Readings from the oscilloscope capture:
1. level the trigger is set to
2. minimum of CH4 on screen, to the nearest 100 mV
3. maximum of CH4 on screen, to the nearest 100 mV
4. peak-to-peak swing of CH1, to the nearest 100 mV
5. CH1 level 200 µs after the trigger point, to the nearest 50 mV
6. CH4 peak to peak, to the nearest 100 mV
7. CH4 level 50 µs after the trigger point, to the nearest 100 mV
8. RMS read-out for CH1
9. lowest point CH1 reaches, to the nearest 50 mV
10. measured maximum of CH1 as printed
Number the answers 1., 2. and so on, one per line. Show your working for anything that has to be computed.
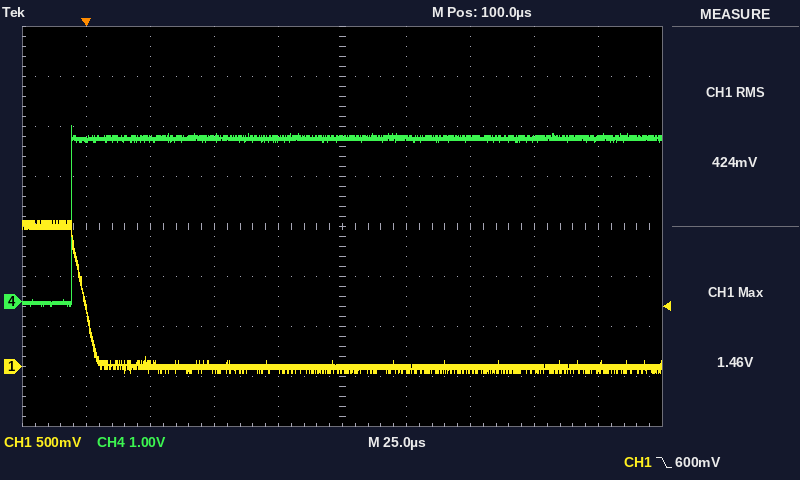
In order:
1. 600 mV
2. -100 mV
3. 3.5 V
4. 1.50 V
5. 0 mV
6. 3.5 V − (-100 mV) = 3.6 V
7. 3.3 V
8. 424 mV
9. -50 mV
10. 1.46 V
